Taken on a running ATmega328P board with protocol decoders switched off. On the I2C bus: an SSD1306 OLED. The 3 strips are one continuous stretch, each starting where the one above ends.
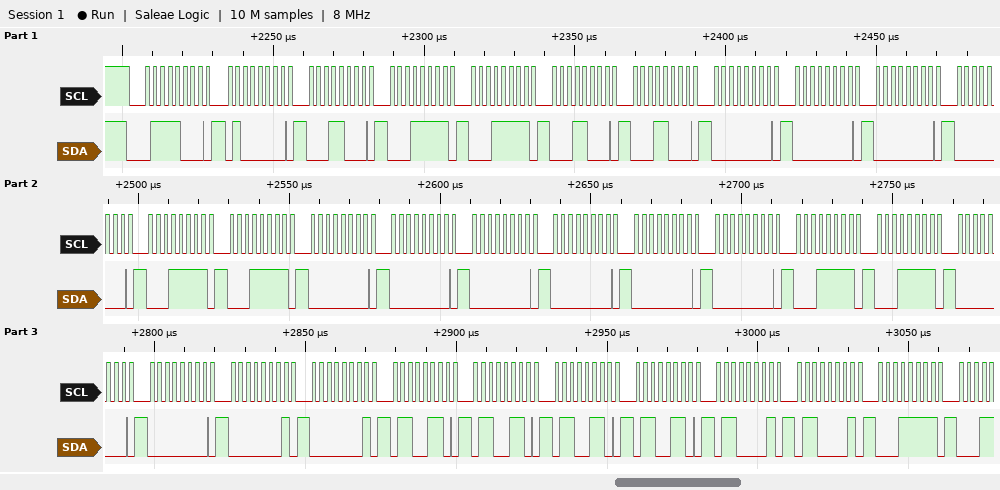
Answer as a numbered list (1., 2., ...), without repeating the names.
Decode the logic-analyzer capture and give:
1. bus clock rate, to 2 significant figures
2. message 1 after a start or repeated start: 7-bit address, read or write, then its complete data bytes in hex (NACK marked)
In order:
1. 400 kHz
2. 0x3C write: 40 18 1F 1F 18 18 00 00 00 00 1F 1F 00 00 00 00 00 00 1F 1F 00 00 01 01 66 66 66 66 61 61 1F
